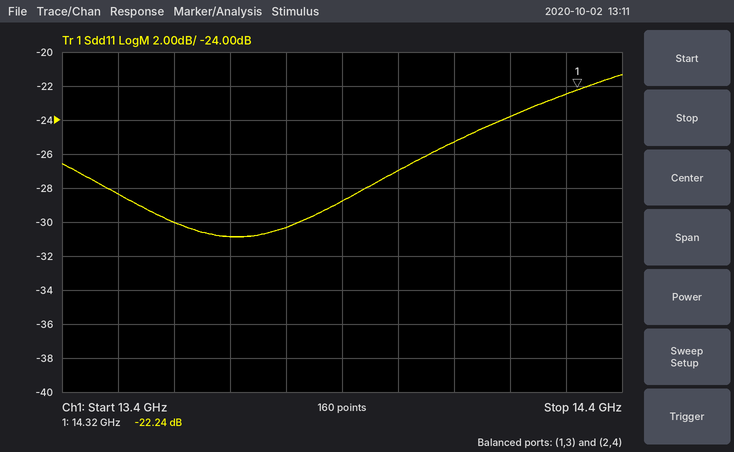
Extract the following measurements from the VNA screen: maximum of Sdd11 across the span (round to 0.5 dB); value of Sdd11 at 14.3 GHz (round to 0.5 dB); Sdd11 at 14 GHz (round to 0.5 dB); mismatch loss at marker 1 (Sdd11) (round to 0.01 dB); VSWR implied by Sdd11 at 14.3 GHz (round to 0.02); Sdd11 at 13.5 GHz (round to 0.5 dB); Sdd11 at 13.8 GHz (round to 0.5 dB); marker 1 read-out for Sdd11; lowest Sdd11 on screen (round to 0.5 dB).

-21.5 dB
-22.5 dB
-27.0 dB
0.03 dB
1.16
-28.5 dB
-30.5 dB
-22.24 dB
-31.0 dB
